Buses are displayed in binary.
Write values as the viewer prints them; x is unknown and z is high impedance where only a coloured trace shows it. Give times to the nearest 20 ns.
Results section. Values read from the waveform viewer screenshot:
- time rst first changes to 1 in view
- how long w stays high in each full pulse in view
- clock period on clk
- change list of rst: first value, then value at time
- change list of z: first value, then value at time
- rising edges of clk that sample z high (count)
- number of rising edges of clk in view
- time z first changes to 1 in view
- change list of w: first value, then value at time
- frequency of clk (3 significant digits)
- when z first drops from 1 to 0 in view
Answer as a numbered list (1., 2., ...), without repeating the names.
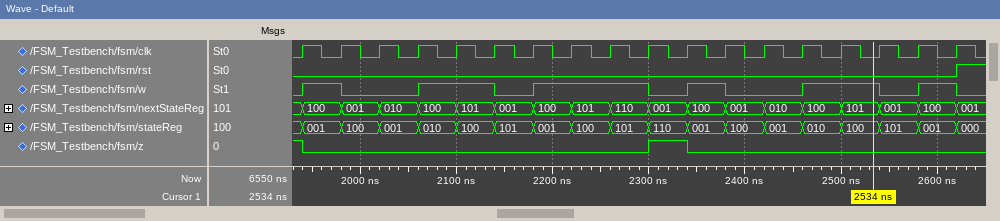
1. 2620 ns
2. 40 ns, 80 ns, 120 ns, 40 ns, 80 ns, 40 ns
3. 40 ns
4. 0, 1 at 2620 ns
5. 1, 0 at 1940 ns, 1 at 2300 ns, 0 at 2340 ns
6. 2
7. 18
8. 2300 ns
9. 0, 1 at 1940 ns, 0 at 1980 ns, 1 at 2060 ns, 0 at 2140 ns, 1 at 2180 ns, 0 at 2300 ns, 1 at 2340 ns, 0 at 2380 ns, 1 at 2460 ns, 0 at 2540 ns, 1 at 2580 ns, 0 at 2620 ns
10. 25.0 MHz
11. 1940 ns
